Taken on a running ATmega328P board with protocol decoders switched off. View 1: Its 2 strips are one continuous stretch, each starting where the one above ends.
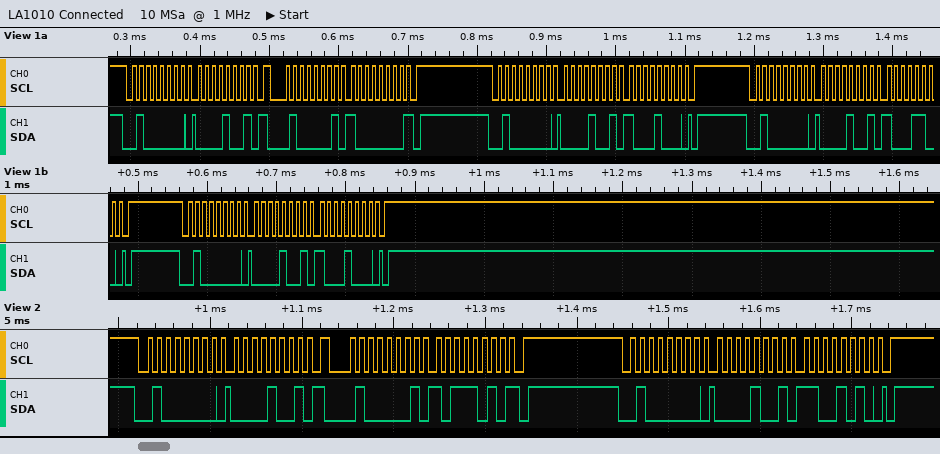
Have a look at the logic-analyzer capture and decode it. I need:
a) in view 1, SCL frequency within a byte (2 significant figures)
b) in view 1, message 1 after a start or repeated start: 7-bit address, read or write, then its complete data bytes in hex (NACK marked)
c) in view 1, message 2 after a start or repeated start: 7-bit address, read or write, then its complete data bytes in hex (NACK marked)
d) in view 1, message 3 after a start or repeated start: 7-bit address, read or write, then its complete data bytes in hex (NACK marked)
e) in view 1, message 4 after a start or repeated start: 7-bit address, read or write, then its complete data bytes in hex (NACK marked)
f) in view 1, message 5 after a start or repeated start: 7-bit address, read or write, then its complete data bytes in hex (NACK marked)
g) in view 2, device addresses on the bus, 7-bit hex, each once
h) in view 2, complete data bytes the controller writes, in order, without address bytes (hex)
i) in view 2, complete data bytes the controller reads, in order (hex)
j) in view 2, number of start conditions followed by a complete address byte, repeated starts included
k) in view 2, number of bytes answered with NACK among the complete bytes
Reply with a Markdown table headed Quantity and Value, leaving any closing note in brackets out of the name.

| Quantity | Value |
|---|---|
| in view 1, SCL frequency within a byte | 100 kHz |
| in view 1, message 1 after a start or repeated start: 7-bit address, read or write, then its complete data bytes in hex | 0x20 write: 09 |
| in view 1, message 2 after a start or repeated start: 7-bit address, read or write, then its complete data bytes in hex | 0x20 read: 80 NACK |
| in view 1, message 3 after a start or repeated start: 7-bit address, read or write, then its complete data bytes in hex | 0x20 write: 09 88 |
| in view 1, message 4 after a start or repeated start: 7-bit address, read or write, then its complete data bytes in hex | 0x20 write: 09 8C |
| in view 1, message 5 after a start or repeated start: 7-bit address, read or write, then its complete data bytes in hex | 0x20 write: 09 88 |
| in view 2, device addresses on the bus, 7-bit hex, each once | 0x20 |
| in view 2, complete data bytes the controller writes, in order, without address bytes | 09 09 CA |
| in view 2, complete data bytes the controller reads, in order | BA |
| in view 2, number of start conditions followed by a complete address byte, repeated starts included | 3 |
| in view 2, number of bytes answered with NACK among the complete bytes | 1 |
